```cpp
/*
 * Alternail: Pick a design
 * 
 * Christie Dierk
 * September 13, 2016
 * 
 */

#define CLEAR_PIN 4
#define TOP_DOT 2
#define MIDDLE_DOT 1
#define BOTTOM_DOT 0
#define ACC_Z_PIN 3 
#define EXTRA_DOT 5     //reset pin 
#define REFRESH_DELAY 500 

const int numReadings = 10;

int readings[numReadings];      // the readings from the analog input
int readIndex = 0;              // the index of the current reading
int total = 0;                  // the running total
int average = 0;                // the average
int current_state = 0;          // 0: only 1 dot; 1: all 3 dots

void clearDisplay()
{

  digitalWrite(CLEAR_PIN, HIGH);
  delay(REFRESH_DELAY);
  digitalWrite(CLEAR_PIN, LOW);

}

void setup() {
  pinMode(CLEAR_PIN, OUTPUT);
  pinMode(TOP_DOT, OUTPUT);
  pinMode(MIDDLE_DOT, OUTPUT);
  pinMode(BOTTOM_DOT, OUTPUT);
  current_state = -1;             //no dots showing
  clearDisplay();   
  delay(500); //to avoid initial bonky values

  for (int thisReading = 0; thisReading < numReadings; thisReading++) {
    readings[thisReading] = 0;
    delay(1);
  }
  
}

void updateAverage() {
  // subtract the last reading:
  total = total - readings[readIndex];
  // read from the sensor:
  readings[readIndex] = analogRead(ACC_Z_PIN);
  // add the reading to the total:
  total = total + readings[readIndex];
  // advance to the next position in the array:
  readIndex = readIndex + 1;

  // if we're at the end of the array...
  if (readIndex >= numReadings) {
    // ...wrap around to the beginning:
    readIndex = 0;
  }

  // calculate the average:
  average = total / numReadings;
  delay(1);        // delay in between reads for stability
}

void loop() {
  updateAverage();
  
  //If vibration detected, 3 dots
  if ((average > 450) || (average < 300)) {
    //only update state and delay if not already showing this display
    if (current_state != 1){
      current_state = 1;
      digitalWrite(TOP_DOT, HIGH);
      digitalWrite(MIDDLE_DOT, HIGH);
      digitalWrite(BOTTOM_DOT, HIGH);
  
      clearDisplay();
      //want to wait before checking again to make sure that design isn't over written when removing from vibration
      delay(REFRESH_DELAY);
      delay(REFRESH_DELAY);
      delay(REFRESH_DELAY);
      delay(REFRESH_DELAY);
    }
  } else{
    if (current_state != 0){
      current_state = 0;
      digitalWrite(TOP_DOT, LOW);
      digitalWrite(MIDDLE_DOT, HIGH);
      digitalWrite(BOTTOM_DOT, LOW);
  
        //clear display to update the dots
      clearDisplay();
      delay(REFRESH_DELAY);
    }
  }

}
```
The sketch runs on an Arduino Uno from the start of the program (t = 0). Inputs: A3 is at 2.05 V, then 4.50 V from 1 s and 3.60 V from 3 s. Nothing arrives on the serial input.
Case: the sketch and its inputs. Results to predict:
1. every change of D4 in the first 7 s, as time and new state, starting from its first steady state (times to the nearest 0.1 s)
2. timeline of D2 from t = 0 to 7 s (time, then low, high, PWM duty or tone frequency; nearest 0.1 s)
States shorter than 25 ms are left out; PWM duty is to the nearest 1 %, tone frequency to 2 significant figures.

0 s high; 0.5 s low; 1 s high; 1.5 s low; 3.5 s high; 4 s low; 4.5 s high; 5 s low
0 s low; 1 s high; 3.5 s low; 4.5 s high
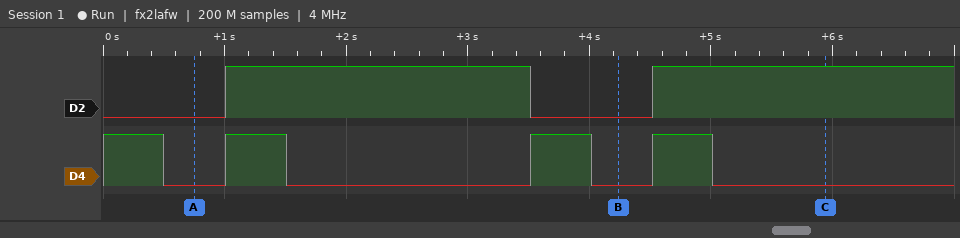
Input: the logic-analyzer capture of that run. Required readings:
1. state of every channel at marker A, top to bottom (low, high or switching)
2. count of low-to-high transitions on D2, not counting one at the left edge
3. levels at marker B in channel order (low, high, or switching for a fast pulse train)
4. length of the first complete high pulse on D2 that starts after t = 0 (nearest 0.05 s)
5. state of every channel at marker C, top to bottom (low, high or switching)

D2 low, D4 low
2
D2 low, D4 low
2.50 s
D2 high, D4 low
